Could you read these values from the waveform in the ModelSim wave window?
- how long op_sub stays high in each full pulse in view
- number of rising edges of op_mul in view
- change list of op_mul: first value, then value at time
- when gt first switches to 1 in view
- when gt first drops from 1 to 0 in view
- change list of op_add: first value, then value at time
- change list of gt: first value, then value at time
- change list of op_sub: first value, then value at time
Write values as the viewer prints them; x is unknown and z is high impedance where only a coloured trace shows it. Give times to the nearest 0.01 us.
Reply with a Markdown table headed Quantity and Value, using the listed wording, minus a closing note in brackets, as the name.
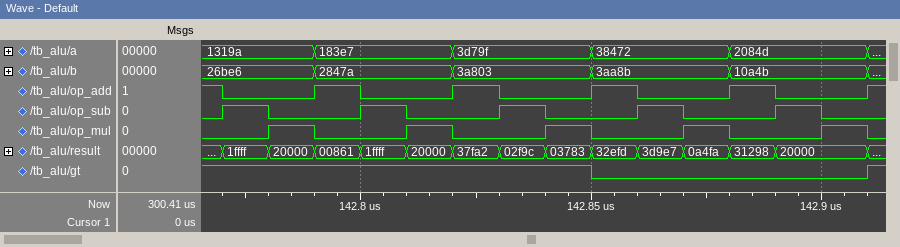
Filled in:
| Quantity | Value |
|---|---|
| how long op_sub stays high in each full pulse in view | 0.01 us, 0.01 us, 0.01 us, 0.01 us, 0.01 us |
| number of rising edges of op_mul in view | 5 |
| change list of op_mul: first value, then value at time | 0, 1 at 142.78 us, 0 at 142.79 us, 1 at 142.81 us, 0 at 142.82 us, 1 at 142.84 us, 0 at 142.85 us, 1 at 142.87 us, 0 at 142.88 us, 1 at 142.9 us, 0 at 142.91 us |
| when gt first switches to 1 in view | 142.91 us |
| when gt first drops from 1 to 0 in view | 142.85 us |
| change list of op_add: first value, then value at time | 1, 0 at 142.77 us, 1 at 142.79 us, 0 at 142.8 us, 1 at 142.82 us, 0 at 142.83 us, 1 at 142.85 us, 0 at 142.86 us, 1 at 142.88 us, 0 at 142.89 us, 1 at 142.91 us |
| change list of gt: first value, then value at time | 1, 0 at 142.85 us, 1 at 142.91 us |
| change list of op_sub: first value, then value at time | 0, 1 at 142.77 us, 0 at 142.78 us, 1 at 142.8 us, 0 at 142.81 us, 1 at 142.83 us, 0 at 142.84 us, 1 at 142.86 us, 0 at 142.87 us, 1 at 142.89 us, 0 at 142.9 us |
